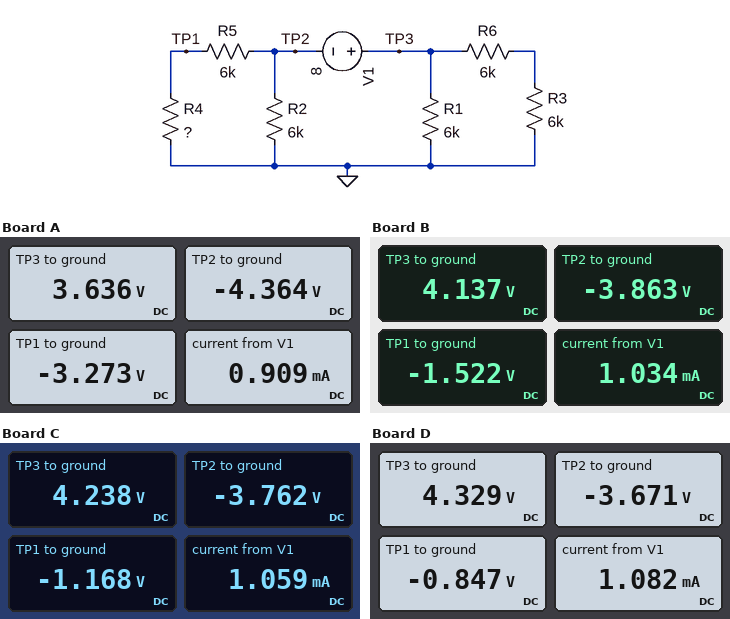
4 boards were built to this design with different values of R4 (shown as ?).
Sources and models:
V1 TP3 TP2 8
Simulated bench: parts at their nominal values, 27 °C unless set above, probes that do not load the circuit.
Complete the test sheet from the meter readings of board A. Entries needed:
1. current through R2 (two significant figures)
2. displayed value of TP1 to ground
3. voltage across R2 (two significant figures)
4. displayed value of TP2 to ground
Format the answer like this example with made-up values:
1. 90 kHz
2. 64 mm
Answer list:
1. 730 µA
2. -3.273 V
3. 4.4 V
4. -4.364 V
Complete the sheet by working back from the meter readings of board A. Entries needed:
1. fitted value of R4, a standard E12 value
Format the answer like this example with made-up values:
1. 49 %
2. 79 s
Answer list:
1. 18 kΩ
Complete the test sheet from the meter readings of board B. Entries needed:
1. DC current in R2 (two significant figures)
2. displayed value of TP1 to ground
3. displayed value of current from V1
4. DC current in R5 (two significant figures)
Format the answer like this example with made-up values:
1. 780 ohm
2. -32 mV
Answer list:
1. 640 µA
2. -1.522 V
3. 1.034 mA
4. 390 µA
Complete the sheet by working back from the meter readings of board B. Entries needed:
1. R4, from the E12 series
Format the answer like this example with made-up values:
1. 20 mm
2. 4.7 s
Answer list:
1. 3.9 kΩ
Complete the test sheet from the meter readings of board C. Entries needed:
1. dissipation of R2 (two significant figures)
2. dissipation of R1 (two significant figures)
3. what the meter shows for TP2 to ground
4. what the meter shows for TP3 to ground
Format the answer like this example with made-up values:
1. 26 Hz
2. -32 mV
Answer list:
1. 2.4 mW
2. 3.0 mW
3. -3.762 V
4. 4.238 V
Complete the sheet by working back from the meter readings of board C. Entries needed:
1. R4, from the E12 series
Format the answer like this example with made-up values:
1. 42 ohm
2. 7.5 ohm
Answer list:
1. 2.7 kΩ
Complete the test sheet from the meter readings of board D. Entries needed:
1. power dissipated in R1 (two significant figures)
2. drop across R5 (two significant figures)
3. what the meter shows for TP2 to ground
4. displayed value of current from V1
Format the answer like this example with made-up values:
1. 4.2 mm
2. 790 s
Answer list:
1. 3.1 mW
2. 2.8 V
3. -3.671 V
4. 1.082 mA
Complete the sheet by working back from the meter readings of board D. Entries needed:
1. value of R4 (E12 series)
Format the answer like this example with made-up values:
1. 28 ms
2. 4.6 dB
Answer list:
1. 1.8 kΩ
